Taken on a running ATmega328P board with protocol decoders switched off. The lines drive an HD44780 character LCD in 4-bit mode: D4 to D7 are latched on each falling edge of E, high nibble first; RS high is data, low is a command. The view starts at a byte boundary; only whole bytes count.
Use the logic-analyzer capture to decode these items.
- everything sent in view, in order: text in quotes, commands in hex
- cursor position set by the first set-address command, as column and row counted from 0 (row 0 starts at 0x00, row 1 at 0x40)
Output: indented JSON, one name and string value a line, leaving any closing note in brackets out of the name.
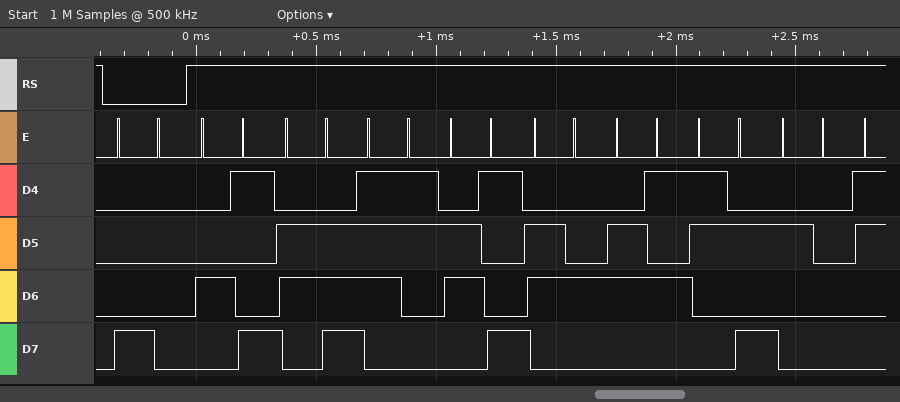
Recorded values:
{
  "everything sent in view, in order: text in quotes, commands in hex": "0x80 \"Inside: \"",
  "cursor position set by the first set-address command, as column and row counted from 0": "column 0, row 0"
}
